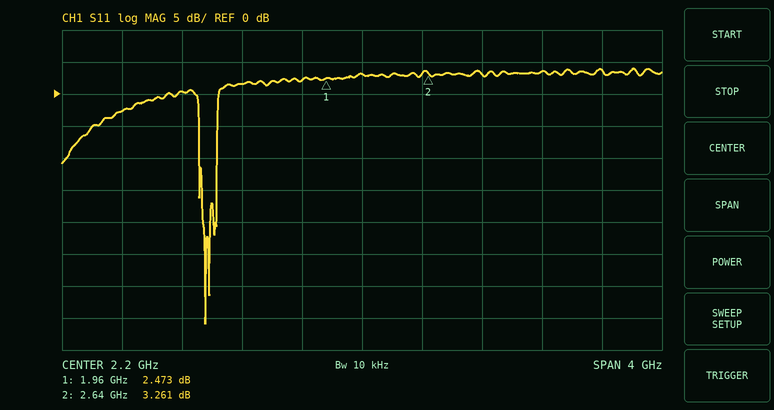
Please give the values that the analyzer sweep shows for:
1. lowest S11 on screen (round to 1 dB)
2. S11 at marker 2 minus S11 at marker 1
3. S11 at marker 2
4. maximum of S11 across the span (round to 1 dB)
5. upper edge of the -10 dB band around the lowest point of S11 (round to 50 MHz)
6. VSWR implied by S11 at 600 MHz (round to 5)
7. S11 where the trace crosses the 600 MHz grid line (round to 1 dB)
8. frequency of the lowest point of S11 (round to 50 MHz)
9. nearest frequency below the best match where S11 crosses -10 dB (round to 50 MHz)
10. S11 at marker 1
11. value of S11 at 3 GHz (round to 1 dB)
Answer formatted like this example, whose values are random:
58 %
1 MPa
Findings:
-36 dB
0.788 dB
3.261 dB
4 dB
1.25 GHz
5
-3 dB
1.15 GHz
1.10 GHz
2.473 dB
3 dB
